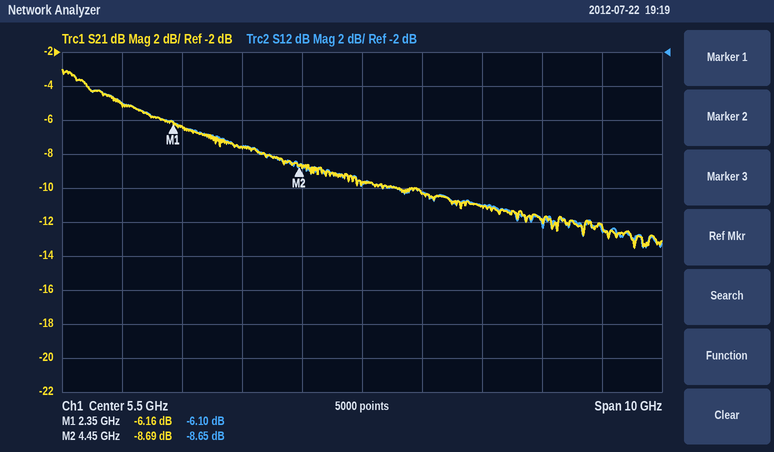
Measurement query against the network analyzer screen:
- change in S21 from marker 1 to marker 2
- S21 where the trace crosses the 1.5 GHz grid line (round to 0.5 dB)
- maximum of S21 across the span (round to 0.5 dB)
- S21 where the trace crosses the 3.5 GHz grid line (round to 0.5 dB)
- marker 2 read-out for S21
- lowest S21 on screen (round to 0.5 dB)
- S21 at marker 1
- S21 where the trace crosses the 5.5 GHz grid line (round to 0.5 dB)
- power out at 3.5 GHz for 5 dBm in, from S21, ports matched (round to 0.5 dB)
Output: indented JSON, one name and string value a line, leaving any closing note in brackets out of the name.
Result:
{
  "change in S21 from marker 1 to marker 2": "-2.53 dB",
  "S21 where the trace crosses the 1.5 GHz grid line": "-5.0 dB",
  "maximum of S21 across the span": "-3.0 dB",
  "S21 where the trace crosses the 3.5 GHz grid line": "-7.5 dB",
  "marker 2 read-out for S21": "-8.69 dB",
  "lowest S21 on screen": "-13.5 dB",
  "S21 at marker 1": "-6.16 dB",
  "S21 where the trace crosses the 5.5 GHz grid line": "-9.5 dB",
  "power out at 3.5 GHz for 5 dBm in, from S21, ports matched": "-2.5 dBm"
}
